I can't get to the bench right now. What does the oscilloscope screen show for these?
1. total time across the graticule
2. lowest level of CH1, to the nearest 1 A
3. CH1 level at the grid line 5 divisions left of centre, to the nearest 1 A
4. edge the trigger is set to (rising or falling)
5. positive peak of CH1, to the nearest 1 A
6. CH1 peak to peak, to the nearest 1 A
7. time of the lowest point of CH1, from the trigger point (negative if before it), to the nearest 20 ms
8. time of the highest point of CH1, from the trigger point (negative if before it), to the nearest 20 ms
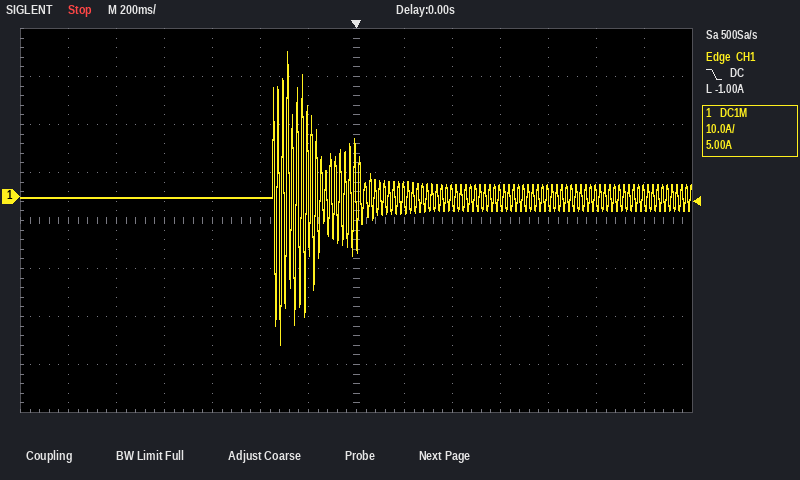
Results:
2.8 s
-31 A
0 A
falling
30 A
61 A
-320 ms
-280 ms
